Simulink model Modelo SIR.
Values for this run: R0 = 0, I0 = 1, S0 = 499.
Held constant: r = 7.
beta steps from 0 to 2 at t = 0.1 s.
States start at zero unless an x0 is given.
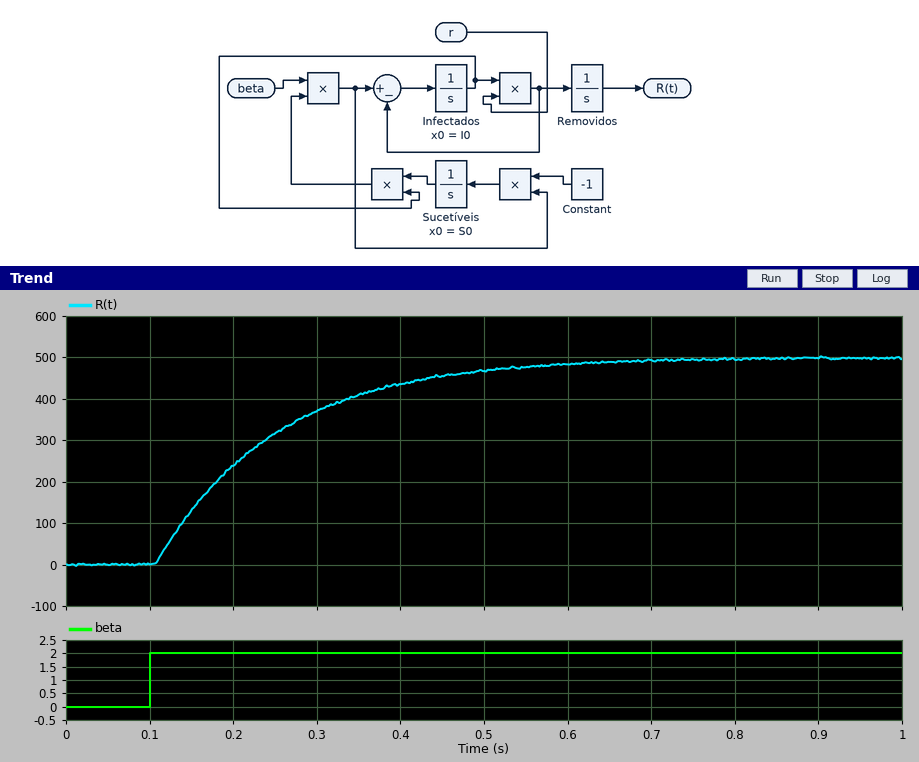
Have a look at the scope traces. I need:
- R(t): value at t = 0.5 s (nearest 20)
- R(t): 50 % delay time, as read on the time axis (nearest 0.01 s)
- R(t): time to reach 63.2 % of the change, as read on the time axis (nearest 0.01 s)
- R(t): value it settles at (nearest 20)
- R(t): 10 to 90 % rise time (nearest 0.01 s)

460
0.21 s
0.25 s
500
0.31 s
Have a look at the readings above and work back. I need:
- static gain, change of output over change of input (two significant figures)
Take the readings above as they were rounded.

250
